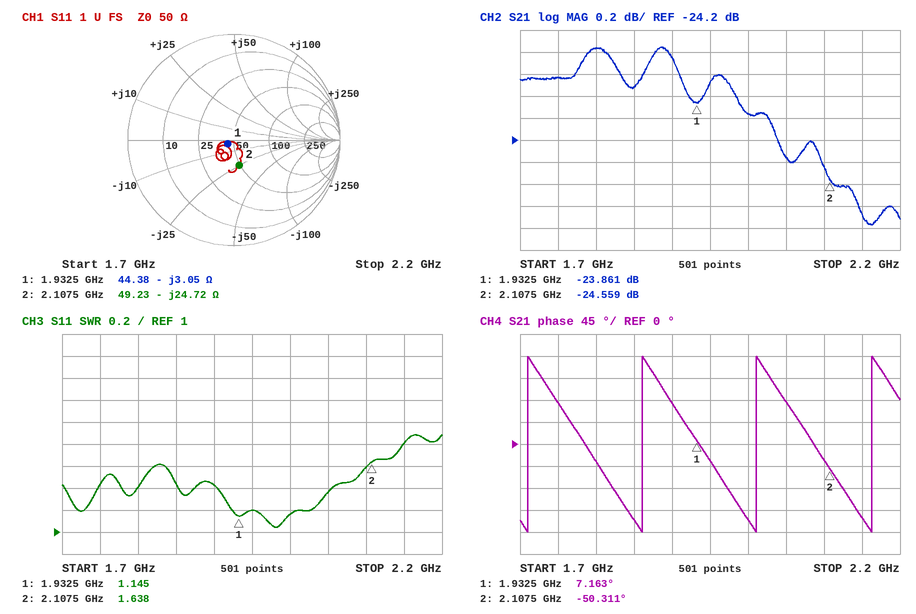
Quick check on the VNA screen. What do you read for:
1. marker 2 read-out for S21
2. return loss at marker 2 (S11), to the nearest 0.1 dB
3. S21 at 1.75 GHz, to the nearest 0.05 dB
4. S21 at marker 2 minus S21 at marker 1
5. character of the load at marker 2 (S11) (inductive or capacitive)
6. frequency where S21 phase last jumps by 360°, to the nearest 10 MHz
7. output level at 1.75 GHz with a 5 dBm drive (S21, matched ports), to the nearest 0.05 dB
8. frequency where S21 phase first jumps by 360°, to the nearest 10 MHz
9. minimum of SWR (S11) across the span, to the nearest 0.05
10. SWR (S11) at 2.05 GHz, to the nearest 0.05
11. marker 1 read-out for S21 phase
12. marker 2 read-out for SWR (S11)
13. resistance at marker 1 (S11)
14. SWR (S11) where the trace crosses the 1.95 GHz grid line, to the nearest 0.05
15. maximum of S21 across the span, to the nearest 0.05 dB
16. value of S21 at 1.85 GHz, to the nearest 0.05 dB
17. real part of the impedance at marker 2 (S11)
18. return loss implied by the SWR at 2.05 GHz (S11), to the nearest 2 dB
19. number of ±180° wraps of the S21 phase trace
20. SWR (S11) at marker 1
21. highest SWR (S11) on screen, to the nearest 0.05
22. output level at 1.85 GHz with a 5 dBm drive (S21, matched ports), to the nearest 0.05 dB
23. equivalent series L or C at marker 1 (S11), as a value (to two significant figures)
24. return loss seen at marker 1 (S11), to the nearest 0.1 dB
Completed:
-24.559 dB
12.3 dB
-23.65 dB
-0.698 dB
capacitive
2.16 GHz
-18.65 dBm
1.71 GHz
1.05
1.35
7.163°
1.638
44.38 Ω
1.20
-23.35 dB
-23.70 dB
49.23 Ω
16 dB
4
1.145
1.90
-18.70 dBm
27 pF
23.4 dB
